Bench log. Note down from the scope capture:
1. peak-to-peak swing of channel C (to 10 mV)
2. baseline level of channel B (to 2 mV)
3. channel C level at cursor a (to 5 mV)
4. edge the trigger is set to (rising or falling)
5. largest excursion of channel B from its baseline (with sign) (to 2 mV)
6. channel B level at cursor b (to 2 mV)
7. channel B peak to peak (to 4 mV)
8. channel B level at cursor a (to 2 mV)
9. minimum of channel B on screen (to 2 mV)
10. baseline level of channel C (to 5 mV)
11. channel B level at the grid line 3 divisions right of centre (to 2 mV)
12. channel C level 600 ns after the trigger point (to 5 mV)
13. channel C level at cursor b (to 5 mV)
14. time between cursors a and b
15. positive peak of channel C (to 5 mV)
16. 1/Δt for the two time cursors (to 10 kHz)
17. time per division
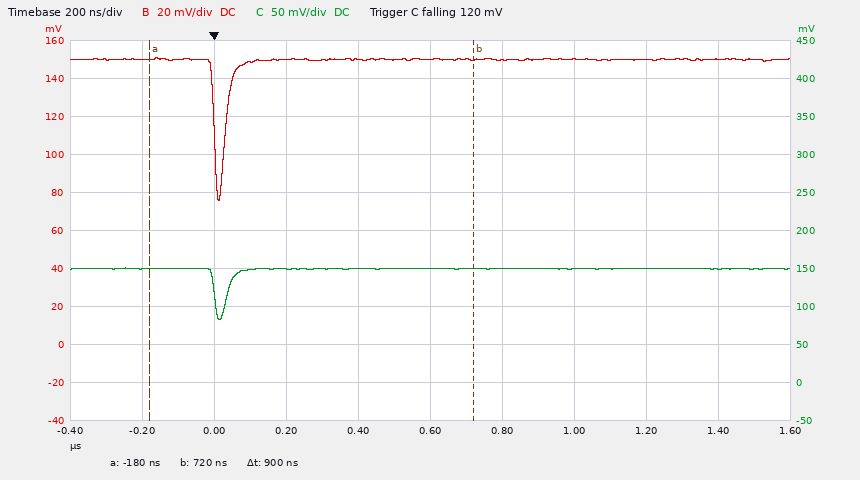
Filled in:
70 mV
150 mV
150 mV
falling
-74 mV
150 mV
76 mV
150 mV
76 mV
150 mV
150 mV
150 mV
150 mV
900 ns
150 mV
1.11 MHz
200 ns
